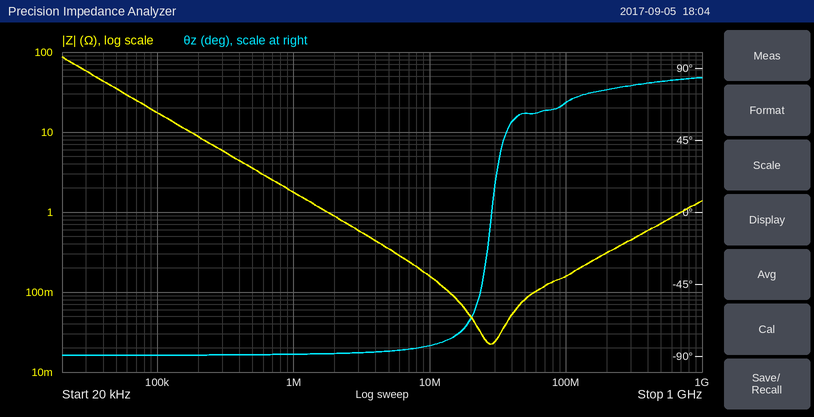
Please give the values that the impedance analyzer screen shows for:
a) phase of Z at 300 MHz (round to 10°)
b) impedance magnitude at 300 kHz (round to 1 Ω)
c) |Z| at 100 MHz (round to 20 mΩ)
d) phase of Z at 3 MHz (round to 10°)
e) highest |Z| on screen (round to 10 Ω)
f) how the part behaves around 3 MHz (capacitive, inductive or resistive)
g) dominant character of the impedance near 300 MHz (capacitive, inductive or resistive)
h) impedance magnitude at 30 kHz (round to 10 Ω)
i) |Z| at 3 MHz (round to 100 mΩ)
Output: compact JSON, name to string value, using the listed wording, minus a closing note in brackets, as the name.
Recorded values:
{"phase of Z at 300 MHz": "80°", "impedance magnitude at 300 kHz": "6 Ω", "|Z| at 100 MHz": "160 mΩ", "phase of Z at 3 MHz": "-90°", "highest |Z| on screen": "90 Ω", "how the part behaves around 3 MHz": "capacitive", "dominant character of the impedance near 300 MHz": "inductive", "impedance magnitude at 30 kHz": "60 Ω", "|Z| at 3 MHz": "600 mΩ"}
